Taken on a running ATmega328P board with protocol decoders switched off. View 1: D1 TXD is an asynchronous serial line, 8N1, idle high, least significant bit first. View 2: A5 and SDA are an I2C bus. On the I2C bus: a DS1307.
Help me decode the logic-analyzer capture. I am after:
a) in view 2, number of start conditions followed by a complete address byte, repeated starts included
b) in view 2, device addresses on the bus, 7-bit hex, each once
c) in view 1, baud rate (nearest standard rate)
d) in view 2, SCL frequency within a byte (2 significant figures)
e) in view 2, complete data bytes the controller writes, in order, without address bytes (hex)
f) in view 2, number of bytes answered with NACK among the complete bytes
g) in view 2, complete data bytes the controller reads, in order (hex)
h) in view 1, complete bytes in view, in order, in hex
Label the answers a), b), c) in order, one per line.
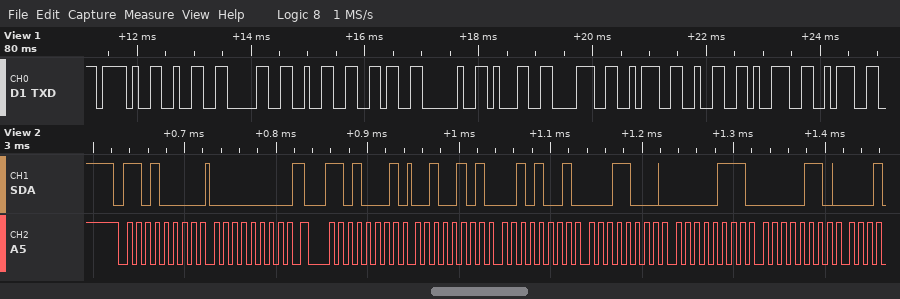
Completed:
a) 2
b) 0x68
c) 9600 baud
d) 100 kHz
e) 00
f) 0
g) 25 29 18 07 06
h) 0x2F 0x32 0x30 0x32 0x36 0x20 0x31 0x38 0x3A 0x32 0x39 0x3A
